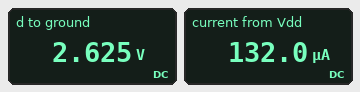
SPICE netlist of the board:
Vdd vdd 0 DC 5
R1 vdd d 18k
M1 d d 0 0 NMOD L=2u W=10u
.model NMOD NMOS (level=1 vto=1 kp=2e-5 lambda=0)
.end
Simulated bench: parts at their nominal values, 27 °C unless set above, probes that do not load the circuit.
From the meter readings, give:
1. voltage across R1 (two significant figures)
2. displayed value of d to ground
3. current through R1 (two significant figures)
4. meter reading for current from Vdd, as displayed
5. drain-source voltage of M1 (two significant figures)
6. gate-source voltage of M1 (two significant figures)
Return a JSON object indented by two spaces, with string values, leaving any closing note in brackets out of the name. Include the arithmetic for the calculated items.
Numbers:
{
  "voltage across R1": "5 V - 2.625 V = 2.4 V",
  "displayed value of d to ground": "2.625 V",
  "current through R1": "(5 V - 2.625 V) / 18 kΩ = 130 µA",
  "meter reading for current from Vdd, as displayed": "132.0 µA",
  "drain-source voltage of M1": "2.625 V = 2.6 V",
  "gate-source voltage of M1": "2.625 V = 2.6 V"
}
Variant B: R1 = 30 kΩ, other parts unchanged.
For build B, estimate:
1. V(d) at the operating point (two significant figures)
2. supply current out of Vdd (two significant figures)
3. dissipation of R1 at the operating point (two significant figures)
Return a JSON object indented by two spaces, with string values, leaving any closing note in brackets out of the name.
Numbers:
{
  "V(d) at the operating point": "2.3 V",
  "supply current out of Vdd": "89 µA",
  "dissipation of R1 at the operating point": "240 µW"
}
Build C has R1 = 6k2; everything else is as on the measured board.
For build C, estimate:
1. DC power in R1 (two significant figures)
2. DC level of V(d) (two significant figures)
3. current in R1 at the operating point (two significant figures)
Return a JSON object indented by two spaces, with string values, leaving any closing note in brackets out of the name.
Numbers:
{
  "DC power in R1": "450 µW",
  "DC level of V(d)": "3.3 V",
  "current in R1 at the operating point": "270 µA"
}
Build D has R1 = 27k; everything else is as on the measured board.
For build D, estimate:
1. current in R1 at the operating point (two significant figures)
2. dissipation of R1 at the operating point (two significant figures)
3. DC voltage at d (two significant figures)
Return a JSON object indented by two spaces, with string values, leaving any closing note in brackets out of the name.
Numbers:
{
  "current in R1 at the operating point": "97 µA",
  "dissipation of R1 at the operating point": "250 µW",
  "DC voltage at d": "2.4 V"
}
